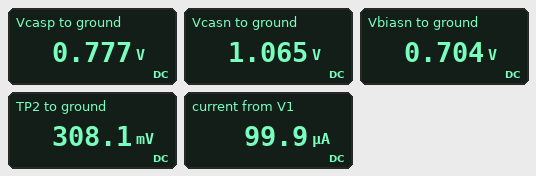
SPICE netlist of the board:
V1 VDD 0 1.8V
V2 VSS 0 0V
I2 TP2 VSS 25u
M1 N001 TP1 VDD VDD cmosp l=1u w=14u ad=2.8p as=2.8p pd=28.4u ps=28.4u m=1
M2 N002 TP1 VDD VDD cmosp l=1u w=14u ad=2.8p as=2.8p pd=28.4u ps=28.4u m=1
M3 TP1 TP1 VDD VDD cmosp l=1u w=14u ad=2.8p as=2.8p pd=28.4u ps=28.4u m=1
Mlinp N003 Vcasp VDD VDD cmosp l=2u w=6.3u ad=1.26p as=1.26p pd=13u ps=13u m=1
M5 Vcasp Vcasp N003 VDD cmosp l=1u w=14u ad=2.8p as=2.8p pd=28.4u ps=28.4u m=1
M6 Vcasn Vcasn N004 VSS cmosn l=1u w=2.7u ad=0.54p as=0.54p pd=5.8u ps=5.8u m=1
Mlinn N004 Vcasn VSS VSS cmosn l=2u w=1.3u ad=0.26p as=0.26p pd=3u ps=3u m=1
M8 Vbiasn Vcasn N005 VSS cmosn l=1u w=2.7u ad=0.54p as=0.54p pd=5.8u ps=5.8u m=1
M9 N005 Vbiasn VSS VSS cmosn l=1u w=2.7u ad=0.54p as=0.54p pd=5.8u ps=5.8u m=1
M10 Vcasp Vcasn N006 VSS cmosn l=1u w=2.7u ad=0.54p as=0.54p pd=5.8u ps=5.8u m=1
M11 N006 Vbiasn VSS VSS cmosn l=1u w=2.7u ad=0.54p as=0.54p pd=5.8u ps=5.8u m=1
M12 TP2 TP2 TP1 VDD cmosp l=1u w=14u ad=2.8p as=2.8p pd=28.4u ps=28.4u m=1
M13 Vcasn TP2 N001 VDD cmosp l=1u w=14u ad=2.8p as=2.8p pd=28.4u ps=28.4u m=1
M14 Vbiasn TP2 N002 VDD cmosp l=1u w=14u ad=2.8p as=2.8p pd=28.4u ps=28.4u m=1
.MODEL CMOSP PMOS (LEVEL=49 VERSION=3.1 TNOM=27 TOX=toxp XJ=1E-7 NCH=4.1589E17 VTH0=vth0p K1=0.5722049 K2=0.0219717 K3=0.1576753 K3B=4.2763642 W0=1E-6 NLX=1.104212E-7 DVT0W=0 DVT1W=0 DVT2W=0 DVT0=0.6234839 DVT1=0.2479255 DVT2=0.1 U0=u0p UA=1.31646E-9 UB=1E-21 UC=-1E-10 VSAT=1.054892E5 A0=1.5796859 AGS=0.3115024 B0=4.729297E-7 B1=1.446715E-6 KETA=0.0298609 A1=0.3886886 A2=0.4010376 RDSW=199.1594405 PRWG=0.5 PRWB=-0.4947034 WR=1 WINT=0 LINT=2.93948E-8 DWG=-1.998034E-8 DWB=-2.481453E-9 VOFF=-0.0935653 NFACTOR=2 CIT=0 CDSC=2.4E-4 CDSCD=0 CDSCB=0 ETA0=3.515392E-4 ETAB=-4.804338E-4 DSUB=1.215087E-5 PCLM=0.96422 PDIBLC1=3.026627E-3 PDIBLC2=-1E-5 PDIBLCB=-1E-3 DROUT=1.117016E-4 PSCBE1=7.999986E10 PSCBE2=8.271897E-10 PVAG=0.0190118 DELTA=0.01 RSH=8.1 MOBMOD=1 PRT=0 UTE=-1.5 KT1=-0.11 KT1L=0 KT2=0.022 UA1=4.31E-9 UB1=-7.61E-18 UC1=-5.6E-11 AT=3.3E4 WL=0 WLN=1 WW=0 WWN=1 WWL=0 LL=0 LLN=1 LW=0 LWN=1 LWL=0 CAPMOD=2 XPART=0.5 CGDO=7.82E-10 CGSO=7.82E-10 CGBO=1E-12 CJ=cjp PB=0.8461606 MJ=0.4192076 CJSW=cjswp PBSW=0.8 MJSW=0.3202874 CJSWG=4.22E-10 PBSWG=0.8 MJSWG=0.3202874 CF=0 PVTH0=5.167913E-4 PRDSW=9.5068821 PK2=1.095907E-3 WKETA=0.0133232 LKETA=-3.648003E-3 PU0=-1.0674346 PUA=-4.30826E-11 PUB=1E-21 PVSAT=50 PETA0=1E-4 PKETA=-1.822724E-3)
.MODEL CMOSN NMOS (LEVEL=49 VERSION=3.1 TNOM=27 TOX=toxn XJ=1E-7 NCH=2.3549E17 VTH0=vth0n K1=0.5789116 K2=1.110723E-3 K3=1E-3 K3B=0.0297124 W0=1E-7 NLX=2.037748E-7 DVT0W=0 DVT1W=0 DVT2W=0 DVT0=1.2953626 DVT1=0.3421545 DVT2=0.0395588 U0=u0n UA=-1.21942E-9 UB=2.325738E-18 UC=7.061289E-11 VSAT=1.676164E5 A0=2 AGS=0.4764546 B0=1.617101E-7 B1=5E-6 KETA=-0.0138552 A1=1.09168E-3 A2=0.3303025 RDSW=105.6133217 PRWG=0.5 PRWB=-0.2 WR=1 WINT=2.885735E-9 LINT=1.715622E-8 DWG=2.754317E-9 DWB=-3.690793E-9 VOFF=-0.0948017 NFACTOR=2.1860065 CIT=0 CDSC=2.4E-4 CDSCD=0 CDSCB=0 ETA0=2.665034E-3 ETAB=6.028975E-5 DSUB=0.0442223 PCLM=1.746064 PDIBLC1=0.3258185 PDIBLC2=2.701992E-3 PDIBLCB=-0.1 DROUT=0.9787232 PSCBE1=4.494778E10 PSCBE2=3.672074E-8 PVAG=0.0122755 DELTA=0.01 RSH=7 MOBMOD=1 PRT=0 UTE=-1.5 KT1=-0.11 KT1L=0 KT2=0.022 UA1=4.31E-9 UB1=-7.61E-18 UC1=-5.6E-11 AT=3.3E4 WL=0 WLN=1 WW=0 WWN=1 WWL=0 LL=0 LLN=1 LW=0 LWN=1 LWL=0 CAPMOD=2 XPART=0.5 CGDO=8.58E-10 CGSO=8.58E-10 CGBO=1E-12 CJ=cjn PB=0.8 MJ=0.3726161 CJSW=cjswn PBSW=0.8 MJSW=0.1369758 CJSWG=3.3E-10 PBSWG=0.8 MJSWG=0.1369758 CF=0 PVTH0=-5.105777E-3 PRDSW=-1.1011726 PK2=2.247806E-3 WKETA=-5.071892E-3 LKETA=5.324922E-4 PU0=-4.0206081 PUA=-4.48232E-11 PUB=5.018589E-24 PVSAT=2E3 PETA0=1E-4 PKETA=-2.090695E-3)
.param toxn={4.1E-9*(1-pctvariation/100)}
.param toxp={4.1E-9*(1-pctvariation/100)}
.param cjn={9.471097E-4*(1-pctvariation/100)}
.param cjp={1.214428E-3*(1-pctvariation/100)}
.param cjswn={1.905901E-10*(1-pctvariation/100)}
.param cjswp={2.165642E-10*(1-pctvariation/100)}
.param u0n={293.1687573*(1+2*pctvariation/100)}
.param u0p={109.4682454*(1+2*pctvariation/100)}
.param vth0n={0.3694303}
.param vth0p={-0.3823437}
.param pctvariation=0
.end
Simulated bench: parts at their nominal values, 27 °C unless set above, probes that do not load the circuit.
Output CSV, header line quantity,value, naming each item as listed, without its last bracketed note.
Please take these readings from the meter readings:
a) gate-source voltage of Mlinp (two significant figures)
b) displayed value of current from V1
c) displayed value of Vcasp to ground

quantity,value
gate-source voltage of Mlinp,-1.0 V
displayed value of current from V1,99.9 µA
displayed value of Vcasp to ground,0.777 V
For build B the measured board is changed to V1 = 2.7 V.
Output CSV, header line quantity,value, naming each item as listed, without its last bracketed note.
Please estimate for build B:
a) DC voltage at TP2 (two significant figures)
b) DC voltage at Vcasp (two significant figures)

quantity,value
DC voltage at TP2,1.2 V
DC voltage at Vcasp,1.7 V
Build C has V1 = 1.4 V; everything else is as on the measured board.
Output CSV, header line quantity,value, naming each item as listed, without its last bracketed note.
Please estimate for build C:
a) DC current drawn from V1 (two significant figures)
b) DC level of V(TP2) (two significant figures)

quantity,value
DC current drawn from V1,99 µA
DC level of V(TP2),-92 mV
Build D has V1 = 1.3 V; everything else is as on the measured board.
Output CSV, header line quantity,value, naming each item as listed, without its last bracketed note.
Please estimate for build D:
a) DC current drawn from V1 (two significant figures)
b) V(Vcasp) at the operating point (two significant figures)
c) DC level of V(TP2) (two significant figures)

quantity,value
DC current drawn from V1,97 µA
V(Vcasp) at the operating point,300 mV
DC level of V(TP2),-190 mV
